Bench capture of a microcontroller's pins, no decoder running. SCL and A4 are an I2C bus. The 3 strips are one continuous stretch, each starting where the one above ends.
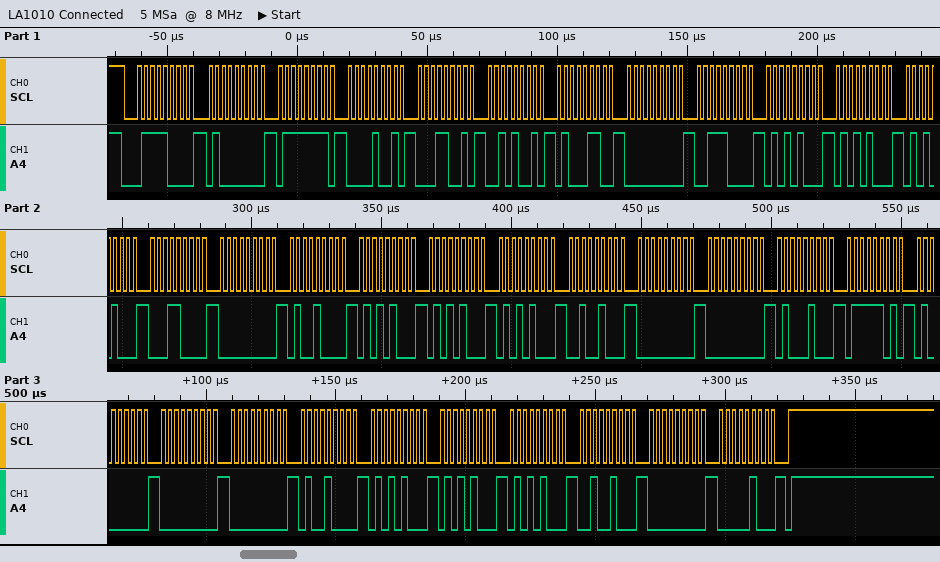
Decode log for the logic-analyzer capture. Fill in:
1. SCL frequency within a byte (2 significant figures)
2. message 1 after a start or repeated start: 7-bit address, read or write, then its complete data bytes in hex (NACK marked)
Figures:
400 kHz
0x3C write: 40 7F 09 19 29 46 00 38 54 54 54 18 00 48 54 54 54 24 00 00 44 7D 40 00 00 48 54 54 54 24 00 04
